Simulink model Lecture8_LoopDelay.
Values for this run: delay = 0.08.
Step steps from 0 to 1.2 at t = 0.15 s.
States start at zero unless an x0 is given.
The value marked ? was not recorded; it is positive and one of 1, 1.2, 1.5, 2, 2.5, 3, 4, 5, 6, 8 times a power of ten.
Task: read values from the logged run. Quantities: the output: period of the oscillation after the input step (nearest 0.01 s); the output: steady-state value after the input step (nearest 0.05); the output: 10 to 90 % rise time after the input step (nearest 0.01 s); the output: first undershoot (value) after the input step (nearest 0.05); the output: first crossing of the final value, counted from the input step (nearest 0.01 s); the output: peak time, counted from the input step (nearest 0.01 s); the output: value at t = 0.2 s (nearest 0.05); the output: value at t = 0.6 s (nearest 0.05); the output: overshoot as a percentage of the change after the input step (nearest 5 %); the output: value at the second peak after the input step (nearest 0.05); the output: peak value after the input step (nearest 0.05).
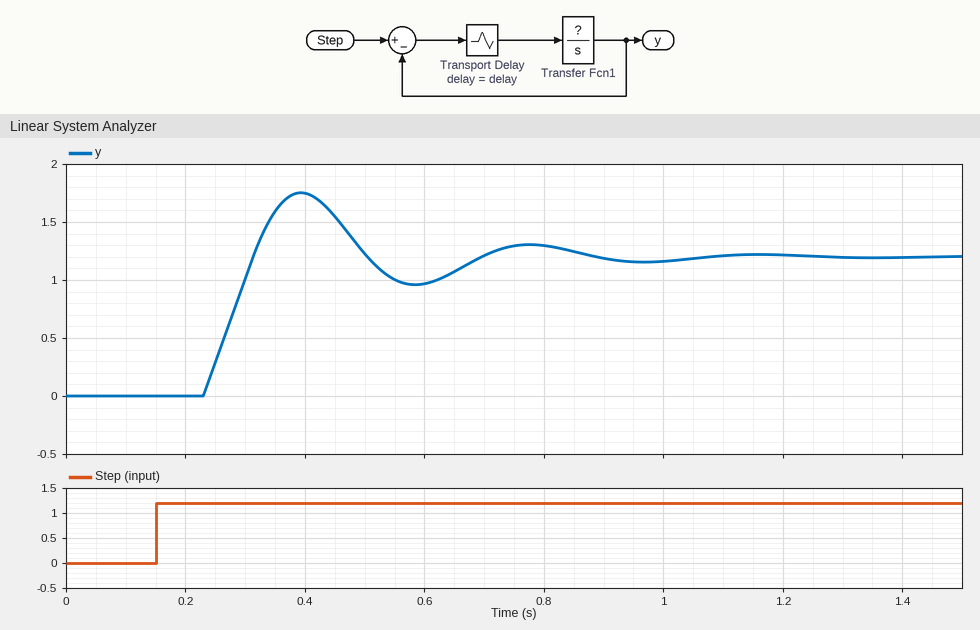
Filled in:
0.38 s
1.20
0.07 s
0.95
0.16 s
0.24 s
0.00
0.95
45 %
1.30
1.75
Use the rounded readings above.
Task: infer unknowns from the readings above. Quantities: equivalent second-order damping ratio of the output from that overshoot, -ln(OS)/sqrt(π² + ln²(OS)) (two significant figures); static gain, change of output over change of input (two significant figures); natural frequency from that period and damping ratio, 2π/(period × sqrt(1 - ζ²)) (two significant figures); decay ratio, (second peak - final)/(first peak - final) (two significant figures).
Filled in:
0.25
1.0
17 rad/s
0.18
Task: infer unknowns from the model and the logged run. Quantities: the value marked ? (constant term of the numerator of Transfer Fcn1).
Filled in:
12
